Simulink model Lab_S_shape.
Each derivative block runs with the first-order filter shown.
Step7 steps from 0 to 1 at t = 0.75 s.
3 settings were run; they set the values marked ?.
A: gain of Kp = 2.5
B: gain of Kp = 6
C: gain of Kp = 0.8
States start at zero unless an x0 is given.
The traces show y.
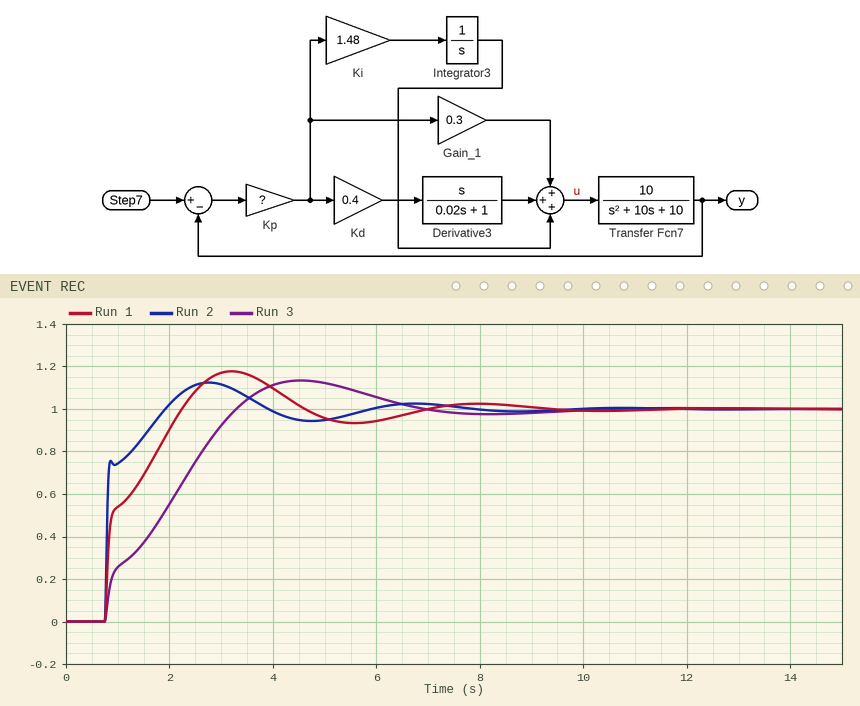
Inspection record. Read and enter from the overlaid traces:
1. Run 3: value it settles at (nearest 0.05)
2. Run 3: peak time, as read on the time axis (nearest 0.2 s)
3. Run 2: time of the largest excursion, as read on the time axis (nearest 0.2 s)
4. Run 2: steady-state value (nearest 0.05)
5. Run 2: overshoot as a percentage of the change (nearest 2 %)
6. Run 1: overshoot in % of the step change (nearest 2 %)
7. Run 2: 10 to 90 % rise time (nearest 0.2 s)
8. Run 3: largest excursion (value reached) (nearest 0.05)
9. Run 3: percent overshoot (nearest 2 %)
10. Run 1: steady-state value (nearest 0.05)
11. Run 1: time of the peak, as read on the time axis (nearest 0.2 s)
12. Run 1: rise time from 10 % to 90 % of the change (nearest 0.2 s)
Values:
1.00
4.6 s
2.8 s
1.00
12 %
18 %
0.8 s
1.15
14 %
1.00
3.2 s
1.2 s
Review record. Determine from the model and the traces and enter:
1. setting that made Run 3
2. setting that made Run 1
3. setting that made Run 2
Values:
C
A
B
